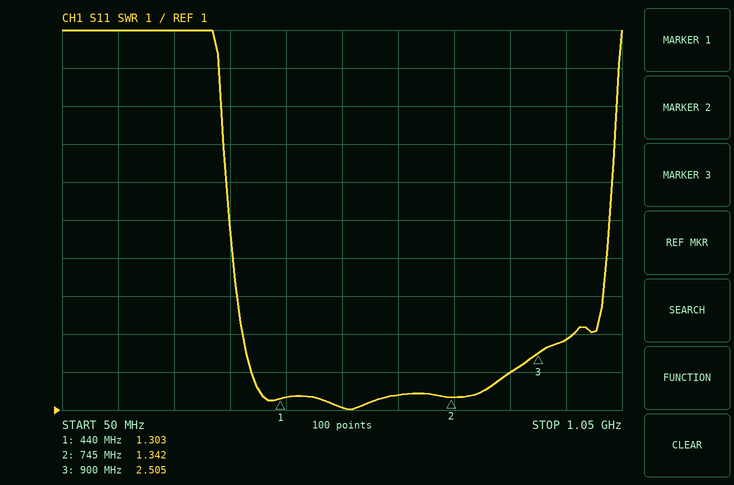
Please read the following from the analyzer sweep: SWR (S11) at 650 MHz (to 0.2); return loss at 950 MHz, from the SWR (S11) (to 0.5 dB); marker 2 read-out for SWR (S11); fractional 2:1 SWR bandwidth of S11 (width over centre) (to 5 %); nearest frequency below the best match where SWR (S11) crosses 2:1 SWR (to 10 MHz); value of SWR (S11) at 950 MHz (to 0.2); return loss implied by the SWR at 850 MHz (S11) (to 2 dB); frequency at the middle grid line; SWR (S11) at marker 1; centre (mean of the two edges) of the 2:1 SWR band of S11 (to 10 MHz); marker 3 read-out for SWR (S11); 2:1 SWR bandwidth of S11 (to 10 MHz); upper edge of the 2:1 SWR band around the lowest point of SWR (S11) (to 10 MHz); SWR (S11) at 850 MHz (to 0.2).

1.4
6.5 dB
1.342
75 %
390 MHz
2.8
10 dB
550 MHz
1.303
620 MHz
2.505
460 MHz
850 MHz
2.0
